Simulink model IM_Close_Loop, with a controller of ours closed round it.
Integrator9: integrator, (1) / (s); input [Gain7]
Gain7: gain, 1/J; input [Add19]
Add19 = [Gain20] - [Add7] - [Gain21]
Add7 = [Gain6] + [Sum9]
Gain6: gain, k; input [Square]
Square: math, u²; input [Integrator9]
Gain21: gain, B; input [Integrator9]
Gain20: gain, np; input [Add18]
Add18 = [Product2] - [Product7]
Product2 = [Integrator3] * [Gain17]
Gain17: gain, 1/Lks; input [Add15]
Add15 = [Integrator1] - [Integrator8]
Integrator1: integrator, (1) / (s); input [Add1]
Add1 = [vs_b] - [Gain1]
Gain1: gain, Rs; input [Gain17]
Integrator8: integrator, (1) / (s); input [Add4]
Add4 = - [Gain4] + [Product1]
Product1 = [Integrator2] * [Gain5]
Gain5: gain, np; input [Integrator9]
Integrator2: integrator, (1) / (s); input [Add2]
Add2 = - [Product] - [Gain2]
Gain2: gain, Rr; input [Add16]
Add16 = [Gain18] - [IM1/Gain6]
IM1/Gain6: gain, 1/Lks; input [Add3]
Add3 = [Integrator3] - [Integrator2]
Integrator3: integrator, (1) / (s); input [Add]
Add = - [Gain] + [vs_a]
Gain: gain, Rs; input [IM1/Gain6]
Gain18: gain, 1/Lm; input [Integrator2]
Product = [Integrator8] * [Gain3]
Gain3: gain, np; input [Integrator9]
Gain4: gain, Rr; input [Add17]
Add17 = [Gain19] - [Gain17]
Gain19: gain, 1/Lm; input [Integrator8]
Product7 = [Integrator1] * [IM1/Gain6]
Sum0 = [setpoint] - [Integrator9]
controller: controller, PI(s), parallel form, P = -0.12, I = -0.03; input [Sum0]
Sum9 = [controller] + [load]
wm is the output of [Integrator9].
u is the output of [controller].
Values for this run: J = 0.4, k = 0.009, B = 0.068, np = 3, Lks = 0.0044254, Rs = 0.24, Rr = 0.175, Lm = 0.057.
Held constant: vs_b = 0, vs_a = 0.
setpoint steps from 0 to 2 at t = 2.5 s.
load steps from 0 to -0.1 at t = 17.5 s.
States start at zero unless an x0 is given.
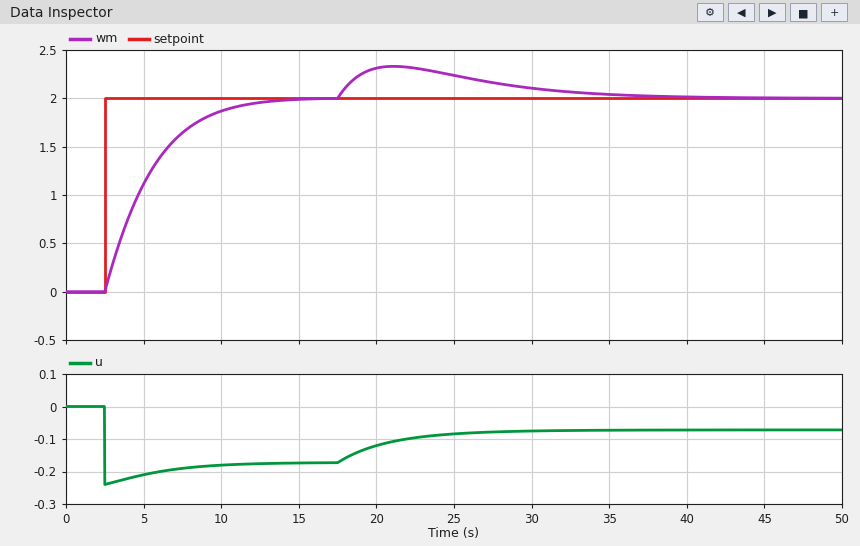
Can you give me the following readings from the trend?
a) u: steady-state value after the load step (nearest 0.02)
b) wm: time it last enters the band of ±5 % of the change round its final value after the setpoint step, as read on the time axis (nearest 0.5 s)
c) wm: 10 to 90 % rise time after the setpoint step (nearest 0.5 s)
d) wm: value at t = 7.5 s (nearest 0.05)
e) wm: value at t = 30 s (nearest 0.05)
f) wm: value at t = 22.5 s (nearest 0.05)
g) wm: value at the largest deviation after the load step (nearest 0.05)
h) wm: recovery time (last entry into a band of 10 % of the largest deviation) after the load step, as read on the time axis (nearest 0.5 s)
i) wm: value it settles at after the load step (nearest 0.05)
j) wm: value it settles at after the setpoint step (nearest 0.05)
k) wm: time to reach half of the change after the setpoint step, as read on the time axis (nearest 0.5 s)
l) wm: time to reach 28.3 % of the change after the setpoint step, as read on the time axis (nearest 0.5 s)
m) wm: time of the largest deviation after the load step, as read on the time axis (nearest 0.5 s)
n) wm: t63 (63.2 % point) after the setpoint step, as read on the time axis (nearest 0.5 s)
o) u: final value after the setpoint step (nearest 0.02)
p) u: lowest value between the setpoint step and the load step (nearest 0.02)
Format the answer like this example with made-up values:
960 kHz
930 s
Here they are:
-0.08
10.5 s
6.0 s
1.65
2.10
2.30
2.35
36.0 s
2.00
2.00
4.5 s
3.5 s
21.0 s
5.5 s
-0.18
-0.24
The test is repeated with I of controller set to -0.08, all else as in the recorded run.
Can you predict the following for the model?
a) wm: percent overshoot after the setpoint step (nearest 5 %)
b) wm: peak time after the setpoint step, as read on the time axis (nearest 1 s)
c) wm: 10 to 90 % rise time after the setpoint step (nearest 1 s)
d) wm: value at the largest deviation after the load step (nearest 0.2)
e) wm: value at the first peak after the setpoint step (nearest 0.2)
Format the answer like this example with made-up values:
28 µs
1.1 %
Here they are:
15 %
9 s
3 s
2.2
2.2
